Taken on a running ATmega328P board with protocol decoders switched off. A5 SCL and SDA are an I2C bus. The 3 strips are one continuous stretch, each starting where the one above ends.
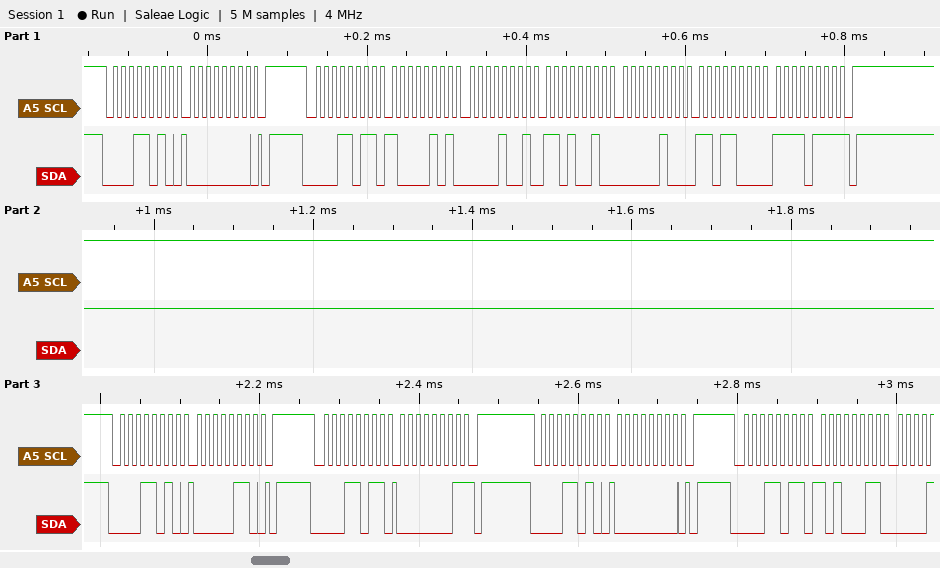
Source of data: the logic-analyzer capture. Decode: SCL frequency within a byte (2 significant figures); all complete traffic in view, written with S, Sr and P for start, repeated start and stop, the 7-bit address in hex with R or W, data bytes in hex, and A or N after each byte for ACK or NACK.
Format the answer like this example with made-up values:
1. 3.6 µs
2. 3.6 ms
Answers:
1. 100 kHz
2. S 0DW A 00 A P S 0DR A 85 A 09 A D2 A 04 A D8 A F7 N P S 0DW A 06 A P S 0DR A 01 N P S 0DW A 00 A P S 0DR A A3 A
